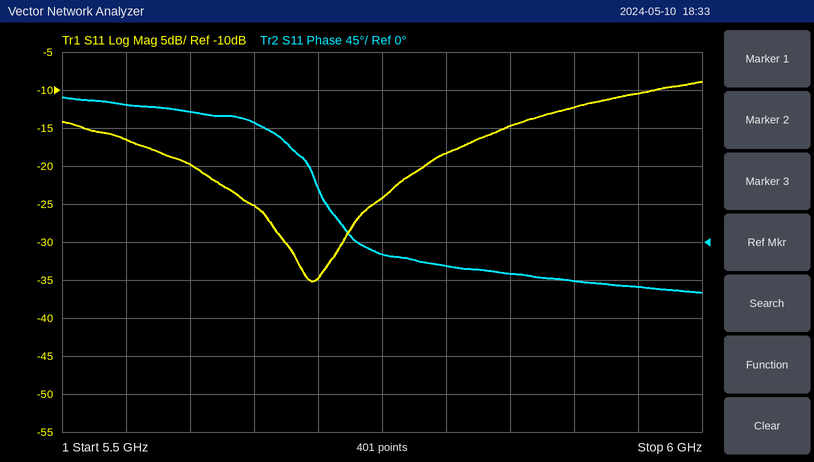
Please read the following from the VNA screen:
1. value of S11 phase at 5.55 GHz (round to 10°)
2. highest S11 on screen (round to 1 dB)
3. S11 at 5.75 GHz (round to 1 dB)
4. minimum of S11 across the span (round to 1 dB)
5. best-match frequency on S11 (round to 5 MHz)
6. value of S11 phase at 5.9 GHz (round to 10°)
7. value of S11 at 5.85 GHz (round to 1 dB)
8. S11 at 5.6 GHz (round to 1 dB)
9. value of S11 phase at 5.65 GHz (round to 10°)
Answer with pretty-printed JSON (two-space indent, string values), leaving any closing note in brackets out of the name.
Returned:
{
  "value of S11 phase at 5.55 GHz": "160°",
  "highest S11 on screen": "-9 dB",
  "S11 at 5.75 GHz": "-24 dB",
  "minimum of S11 across the span": "-35 dB",
  "best-match frequency on S11": "5.695 GHz",
  "value of S11 phase at 5.9 GHz": "-50°",
  "value of S11 at 5.85 GHz": "-15 dB",
  "S11 at 5.6 GHz": "-20 dB",
  "value of S11 phase at 5.65 GHz": "140°"
}
